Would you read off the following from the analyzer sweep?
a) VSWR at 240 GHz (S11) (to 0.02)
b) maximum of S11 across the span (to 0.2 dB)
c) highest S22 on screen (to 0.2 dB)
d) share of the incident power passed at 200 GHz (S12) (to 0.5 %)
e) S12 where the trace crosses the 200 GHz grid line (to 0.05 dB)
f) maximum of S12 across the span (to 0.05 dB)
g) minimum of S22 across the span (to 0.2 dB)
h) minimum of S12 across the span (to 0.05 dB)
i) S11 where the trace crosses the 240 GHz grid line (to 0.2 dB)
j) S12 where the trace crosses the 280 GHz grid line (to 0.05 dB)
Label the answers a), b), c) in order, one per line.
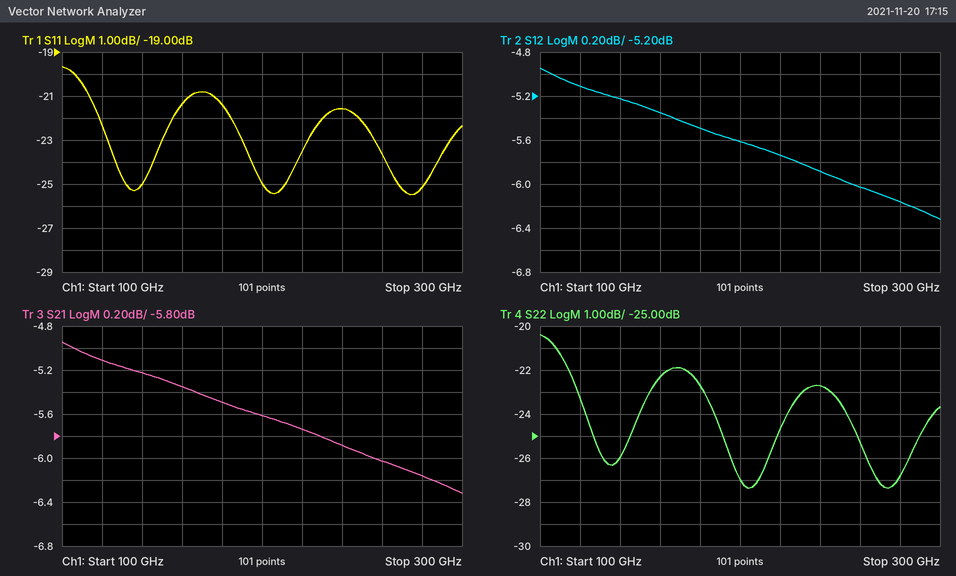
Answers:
a) 1.18
b) -19.6 dB
c) -20.4 dB
d) 27.5 %
e) -5.60 dB
f) -4.95 dB
g) -27.4 dB
h) -6.30 dB
i) -21.6 dB
j) -6.15 dB
